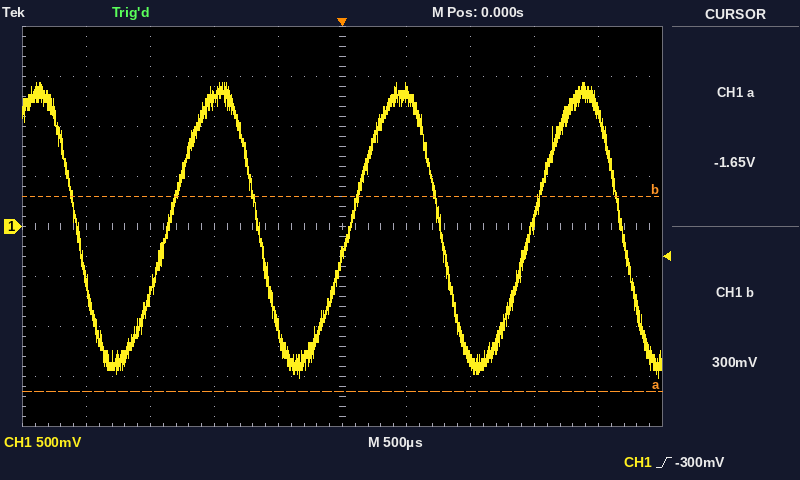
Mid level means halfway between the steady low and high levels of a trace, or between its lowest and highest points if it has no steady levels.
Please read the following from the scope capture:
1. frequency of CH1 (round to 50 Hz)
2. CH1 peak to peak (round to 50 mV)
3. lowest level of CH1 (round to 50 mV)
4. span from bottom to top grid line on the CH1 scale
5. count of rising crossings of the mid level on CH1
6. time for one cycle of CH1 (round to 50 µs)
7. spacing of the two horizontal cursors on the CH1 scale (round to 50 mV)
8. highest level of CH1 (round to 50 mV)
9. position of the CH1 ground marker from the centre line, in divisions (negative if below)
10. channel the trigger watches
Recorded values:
700 Hz
2.95 V
-1.50 V
4 V
3
1.40 ms
1.95 V
1.45 V
0.0 div
CH1
